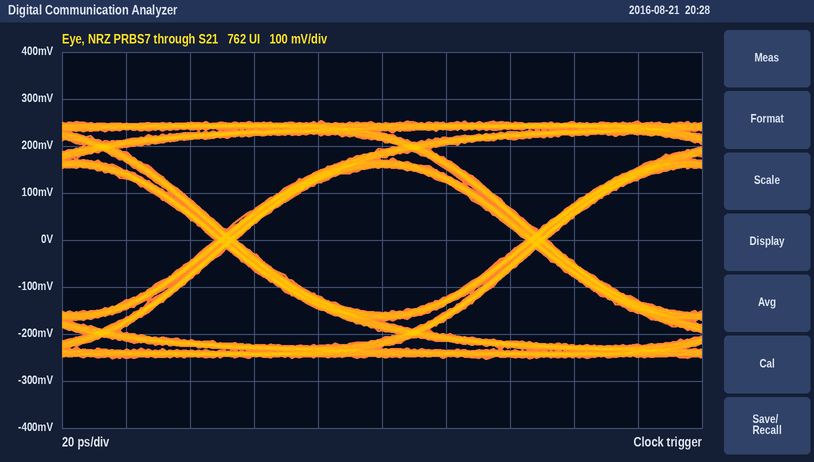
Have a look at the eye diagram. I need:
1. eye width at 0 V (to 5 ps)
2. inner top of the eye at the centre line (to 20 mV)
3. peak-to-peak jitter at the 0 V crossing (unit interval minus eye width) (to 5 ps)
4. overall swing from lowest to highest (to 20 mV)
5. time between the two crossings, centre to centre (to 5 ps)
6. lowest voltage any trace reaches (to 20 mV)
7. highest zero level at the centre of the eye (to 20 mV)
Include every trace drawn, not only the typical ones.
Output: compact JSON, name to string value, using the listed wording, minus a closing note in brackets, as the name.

{"eye width at 0 V": "90 ps", "inner top of the eye at the centre line": "160 mV", "peak-to-peak jitter at the 0 V crossing (unit interval minus eye width)": "5 ps", "overall swing from lowest to highest": "500 mV", "time between the two crossings, centre to centre": "95 ps", "lowest voltage any trace reaches": "-260 mV", "highest zero level at the centre of the eye": "-160 mV"}
